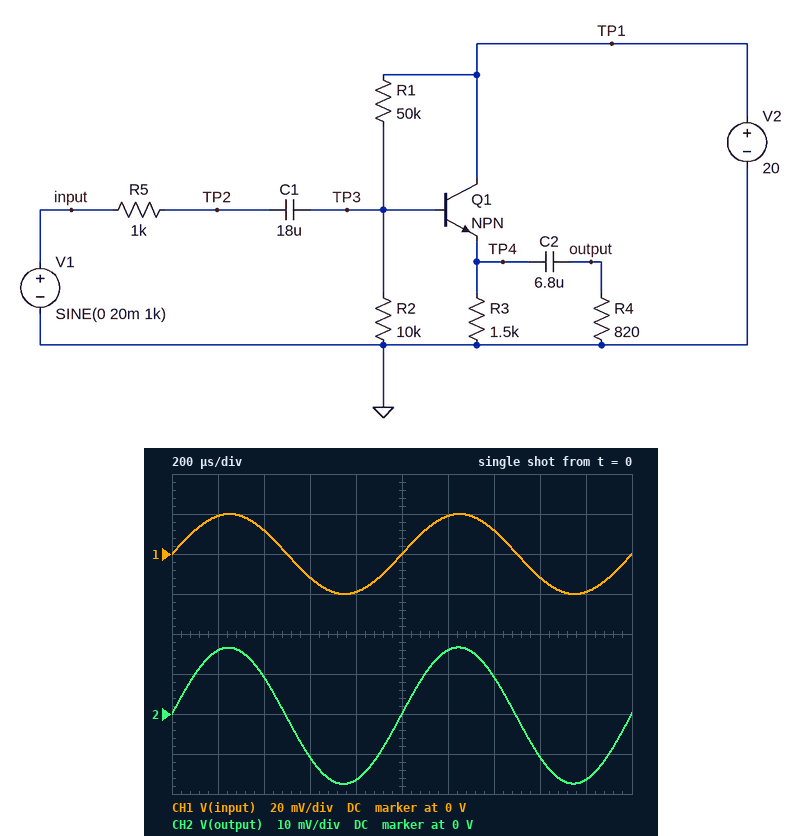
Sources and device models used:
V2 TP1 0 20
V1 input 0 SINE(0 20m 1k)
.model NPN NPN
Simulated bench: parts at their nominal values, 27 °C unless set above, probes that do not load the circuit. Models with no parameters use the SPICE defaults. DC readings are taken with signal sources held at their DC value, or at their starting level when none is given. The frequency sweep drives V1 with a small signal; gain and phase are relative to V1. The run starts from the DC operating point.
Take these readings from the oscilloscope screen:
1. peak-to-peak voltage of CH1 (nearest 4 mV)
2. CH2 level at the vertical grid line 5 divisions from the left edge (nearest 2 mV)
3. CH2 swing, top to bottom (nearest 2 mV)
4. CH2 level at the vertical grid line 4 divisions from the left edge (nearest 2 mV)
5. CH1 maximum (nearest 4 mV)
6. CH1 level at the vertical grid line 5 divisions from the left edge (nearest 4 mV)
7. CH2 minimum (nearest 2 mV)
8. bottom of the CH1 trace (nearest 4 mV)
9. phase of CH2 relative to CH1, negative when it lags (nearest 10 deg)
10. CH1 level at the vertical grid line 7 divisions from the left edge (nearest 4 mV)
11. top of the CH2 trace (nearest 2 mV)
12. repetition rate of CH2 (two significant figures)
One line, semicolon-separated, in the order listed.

40 mV; 0 V; 34 mV; -16 mV; 20 mV; 0 V; -18 mV; -20 mV; 0 deg; 12 mV; 16 mV; 1.0 kHz
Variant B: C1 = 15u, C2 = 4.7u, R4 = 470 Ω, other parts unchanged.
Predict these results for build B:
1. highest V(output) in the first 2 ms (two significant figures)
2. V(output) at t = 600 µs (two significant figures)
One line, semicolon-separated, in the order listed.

16 mV; -12 mV
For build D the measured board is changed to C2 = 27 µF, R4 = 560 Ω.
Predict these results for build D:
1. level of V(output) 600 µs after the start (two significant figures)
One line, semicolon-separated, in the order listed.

-10 mV
